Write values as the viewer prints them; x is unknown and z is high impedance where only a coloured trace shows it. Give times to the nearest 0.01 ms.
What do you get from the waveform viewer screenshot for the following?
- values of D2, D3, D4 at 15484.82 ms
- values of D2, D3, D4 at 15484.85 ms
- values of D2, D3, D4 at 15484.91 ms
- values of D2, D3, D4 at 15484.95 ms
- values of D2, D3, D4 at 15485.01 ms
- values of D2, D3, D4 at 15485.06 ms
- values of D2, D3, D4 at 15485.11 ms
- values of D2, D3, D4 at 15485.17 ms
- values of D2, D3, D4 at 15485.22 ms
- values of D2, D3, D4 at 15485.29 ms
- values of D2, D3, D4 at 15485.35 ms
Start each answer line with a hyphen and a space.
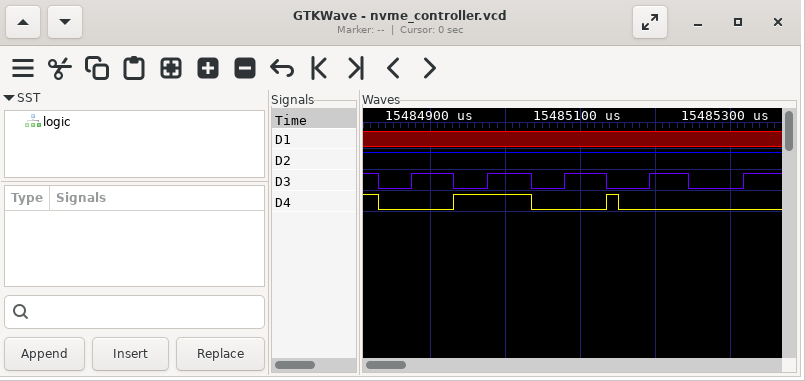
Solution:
- D2=1, D3=1, D4=1
- D2=1, D3=0, D4=0
- D2=1, D3=1, D4=0
- D2=1, D3=0, D4=1
- D2=1, D3=1, D4=1
- D2=1, D3=0, D4=0
- D2=1, D3=1, D4=0
- D2=1, D3=0, D4=0
- D2=1, D3=1, D4=0
- D2=1, D3=0, D4=0
- D2=1, D3=1, D4=0
